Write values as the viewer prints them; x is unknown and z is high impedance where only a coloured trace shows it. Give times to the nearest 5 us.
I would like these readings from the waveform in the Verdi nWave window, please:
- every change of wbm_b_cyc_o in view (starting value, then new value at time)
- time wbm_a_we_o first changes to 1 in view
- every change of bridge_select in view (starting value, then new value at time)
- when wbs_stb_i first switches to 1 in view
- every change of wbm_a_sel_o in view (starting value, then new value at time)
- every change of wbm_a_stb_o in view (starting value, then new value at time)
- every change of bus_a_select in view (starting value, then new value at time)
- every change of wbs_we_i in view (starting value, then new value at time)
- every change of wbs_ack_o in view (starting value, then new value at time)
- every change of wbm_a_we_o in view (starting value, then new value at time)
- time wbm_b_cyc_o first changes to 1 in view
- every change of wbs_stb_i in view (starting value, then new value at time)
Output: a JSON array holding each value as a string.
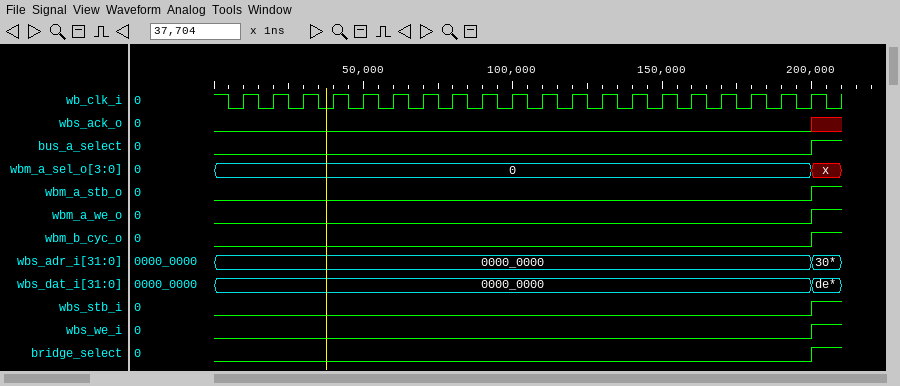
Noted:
["0, 1 at 200 us", "200 us", "0, 1 at 200 us", "200 us", "0, x at 200 us", "0, 1 at 200 us", "0, 1 at 200 us", "0, 1 at 200 us", "0, x at 200 us", "0, 1 at 200 us", "200 us", "0, 1 at 200 us"]
